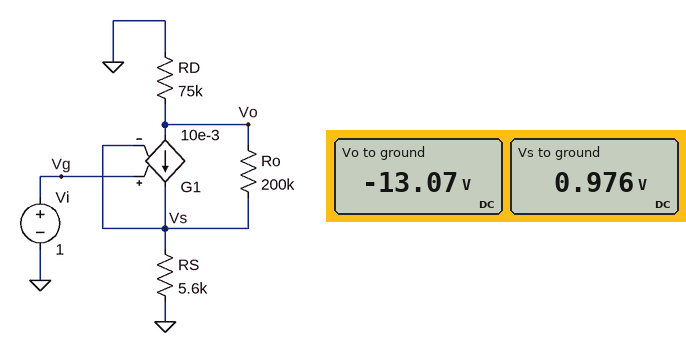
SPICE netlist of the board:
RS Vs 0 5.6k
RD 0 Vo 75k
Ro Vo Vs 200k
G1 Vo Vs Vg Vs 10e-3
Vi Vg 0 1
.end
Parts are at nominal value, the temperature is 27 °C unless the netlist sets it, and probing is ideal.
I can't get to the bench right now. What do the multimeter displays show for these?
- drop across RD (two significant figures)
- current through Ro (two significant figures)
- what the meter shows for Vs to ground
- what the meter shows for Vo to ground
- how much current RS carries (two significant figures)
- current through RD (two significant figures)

13 V
70 µA
0.976 V
-13.07 V
170 µA
170 µA
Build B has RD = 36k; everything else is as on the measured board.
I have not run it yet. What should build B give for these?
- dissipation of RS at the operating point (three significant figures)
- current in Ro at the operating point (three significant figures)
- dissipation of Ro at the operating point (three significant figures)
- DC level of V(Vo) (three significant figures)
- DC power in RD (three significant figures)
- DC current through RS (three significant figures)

171 µW
36.4 µA
264 µW
-6.29 V
1.10 mW
175 µA
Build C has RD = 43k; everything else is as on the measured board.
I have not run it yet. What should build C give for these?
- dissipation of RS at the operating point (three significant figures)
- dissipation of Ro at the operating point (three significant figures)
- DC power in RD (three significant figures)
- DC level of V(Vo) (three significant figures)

171 µW
360 µW
1.31 mW
-7.51 V
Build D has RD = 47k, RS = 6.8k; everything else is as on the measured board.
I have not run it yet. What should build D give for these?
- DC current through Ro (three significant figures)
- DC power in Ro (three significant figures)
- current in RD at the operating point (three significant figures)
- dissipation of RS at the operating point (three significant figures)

38.8 µA
302 µW
144 µA
142 µW
